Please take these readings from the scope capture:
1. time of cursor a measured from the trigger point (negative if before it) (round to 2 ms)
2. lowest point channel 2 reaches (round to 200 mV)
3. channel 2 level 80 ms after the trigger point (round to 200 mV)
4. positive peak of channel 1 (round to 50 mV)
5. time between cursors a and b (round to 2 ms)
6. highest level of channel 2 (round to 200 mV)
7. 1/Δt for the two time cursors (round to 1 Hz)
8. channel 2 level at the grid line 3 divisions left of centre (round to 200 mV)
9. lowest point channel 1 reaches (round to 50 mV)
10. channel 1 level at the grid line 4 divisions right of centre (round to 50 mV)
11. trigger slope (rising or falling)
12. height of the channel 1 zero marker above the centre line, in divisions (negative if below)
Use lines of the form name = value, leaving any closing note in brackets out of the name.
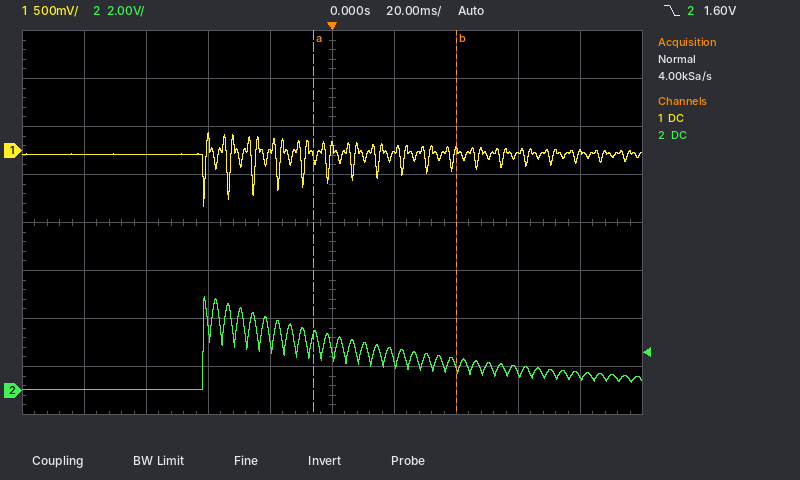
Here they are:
time of cursor a measured from the trigger point (negative if before it) = -6 ms
lowest point channel 2 reaches = 0.0 V
channel 2 level 80 ms after the trigger point = 600 mV
positive peak of channel 1 = 200 mV
time between cursors a and b = 46 ms
highest level of channel 2 = 4.0 V
1/Δt for the two time cursors = 22 Hz
channel 2 level at the grid line 3 divisions left of centre = 0.0 V
lowest point channel 1 reaches = -600 mV
channel 1 level at the grid line 4 divisions right of centre = -50 mV
trigger slope = falling
height of the channel 1 zero marker above the centre line, in divisions = +1.5 div
